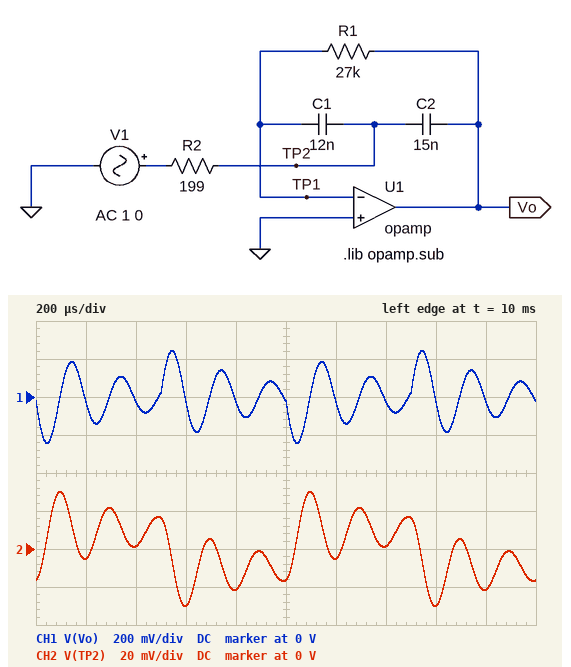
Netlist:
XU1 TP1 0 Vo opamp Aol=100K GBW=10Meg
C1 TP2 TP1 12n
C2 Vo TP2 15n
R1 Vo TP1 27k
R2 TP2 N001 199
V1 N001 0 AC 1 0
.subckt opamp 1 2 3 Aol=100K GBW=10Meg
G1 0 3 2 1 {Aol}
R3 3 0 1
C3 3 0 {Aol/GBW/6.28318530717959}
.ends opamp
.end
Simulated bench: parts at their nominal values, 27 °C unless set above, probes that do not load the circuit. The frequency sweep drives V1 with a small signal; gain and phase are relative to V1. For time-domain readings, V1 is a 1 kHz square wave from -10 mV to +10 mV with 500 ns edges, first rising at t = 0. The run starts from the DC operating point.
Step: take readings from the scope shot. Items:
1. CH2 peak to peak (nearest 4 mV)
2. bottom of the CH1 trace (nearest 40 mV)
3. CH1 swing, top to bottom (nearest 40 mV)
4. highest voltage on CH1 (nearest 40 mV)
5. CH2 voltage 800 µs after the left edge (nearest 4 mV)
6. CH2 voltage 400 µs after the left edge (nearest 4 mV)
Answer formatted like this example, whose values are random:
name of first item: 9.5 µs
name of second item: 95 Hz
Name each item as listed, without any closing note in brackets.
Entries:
CH2 peak to peak: 60 mV
bottom of the CH1 trace: -240 mV
CH1 swing, top to bottom: 480 mV
highest voltage on CH1: 240 mV
CH2 voltage 800 µs after the left edge: -20 mV
CH2 voltage 400 µs after the left edge: 0 V
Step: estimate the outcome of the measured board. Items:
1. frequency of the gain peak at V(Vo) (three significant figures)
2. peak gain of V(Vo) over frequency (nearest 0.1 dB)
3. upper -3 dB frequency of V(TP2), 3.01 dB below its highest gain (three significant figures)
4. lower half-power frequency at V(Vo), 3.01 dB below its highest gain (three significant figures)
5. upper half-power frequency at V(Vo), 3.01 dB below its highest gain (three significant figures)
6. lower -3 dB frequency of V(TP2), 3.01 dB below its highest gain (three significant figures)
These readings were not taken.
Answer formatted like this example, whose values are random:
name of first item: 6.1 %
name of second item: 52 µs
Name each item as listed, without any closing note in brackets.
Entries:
frequency of the gain peak at V(Vo): 5.10 kHz
peak gain of V(Vo) over frequency: 35.6 dB
upper -3 dB frequency of V(TP2), 3.01 dB below its highest gain: 5.49 kHz
lower half-power frequency at V(Vo), 3.01 dB below its highest gain: 4.68 kHz
upper half-power frequency at V(Vo), 3.01 dB below its highest gain: 5.56 kHz
lower -3 dB frequency of V(TP2), 3.01 dB below its highest gain: 4.60 kHz
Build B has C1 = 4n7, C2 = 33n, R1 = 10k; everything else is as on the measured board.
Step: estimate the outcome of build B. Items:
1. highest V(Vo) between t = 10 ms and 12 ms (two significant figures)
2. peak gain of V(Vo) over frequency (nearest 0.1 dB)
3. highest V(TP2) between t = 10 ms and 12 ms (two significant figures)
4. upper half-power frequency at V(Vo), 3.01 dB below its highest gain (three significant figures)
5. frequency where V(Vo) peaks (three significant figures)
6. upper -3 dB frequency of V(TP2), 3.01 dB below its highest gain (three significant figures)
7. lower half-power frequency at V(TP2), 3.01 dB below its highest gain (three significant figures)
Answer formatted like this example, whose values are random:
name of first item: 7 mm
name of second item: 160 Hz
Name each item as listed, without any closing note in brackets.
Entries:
highest V(Vo) between t = 10 ms and 12 ms: 40 mV
peak gain of V(Vo) over frequency: 15.9 dB
highest V(TP2) between t = 10 ms and 12 ms: 20 mV
upper half-power frequency at V(Vo), 3.01 dB below its highest gain: 11.2 kHz
frequency where V(Vo) peaks: 9.05 kHz
upper -3 dB frequency of V(TP2), 3.01 dB below its highest gain: 10.4 kHz
lower half-power frequency at V(TP2), 3.01 dB below its highest gain: 6.34 kHz
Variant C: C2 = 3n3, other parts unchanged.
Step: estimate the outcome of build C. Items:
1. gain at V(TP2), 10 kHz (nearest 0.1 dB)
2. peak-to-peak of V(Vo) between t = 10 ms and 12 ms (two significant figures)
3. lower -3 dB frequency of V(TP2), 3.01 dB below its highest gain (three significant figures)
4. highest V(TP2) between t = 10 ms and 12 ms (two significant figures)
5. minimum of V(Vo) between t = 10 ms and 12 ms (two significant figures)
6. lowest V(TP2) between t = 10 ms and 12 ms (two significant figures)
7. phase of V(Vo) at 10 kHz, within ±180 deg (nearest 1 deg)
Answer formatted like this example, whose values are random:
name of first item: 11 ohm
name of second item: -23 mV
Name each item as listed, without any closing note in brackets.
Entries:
gain at V(TP2), 10 kHz: 12.3 dB
peak-to-peak of V(Vo) between t = 10 ms and 12 ms: 770 mV
lower -3 dB frequency of V(TP2), 3.01 dB below its highest gain: 9.47 kHz
highest V(TP2) between t = 10 ms and 12 ms: 24 mV
minimum of V(Vo) between t = 10 ms and 12 ms: -380 mV
lowest V(TP2) between t = 10 ms and 12 ms: -24 mV
phase of V(Vo) at 10 kHz, within ±180 deg: -144 deg
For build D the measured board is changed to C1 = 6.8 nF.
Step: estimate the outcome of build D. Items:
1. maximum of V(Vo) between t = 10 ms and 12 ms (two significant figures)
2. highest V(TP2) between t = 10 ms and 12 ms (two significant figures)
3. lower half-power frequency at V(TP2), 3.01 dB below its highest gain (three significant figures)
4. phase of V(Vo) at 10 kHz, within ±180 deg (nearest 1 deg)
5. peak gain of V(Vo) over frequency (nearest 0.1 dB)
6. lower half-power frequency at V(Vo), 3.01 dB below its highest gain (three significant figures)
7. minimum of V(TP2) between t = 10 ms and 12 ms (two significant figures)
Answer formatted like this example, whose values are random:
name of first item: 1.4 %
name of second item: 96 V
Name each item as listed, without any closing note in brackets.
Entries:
maximum of V(Vo) between t = 10 ms and 12 ms: 150 mV
highest V(TP2) between t = 10 ms and 12 ms: 26 mV
lower half-power frequency at V(TP2), 3.01 dB below its highest gain: 6.06 kHz
phase of V(Vo) at 10 kHz, within ±180 deg: 103 deg
peak gain of V(Vo) over frequency: 32.5 dB
lower half-power frequency at V(Vo), 3.01 dB below its highest gain: 6.18 kHz
minimum of V(TP2) between t = 10 ms and 12 ms: -26 mV
